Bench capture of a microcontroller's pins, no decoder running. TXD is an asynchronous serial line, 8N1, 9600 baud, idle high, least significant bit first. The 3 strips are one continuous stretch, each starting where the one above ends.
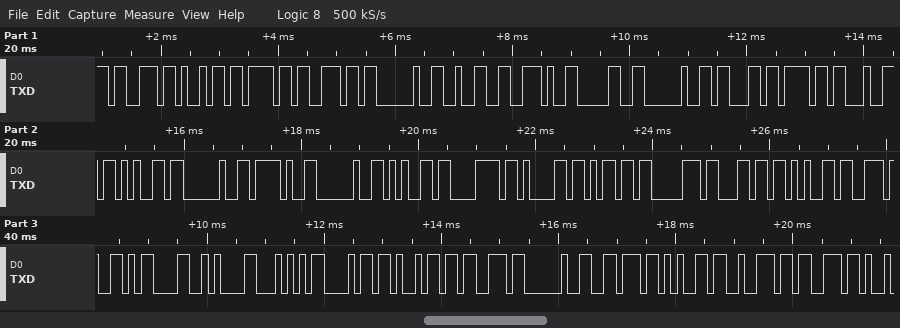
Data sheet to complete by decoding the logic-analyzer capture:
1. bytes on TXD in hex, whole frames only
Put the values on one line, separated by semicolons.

0x73 0x69 0x6F 0x6E 0x20 0x32 0x2E 0x30 0x20 0x63 0x6F 0x64 0x65 0x20 0x2F 0x20 0x65 0x78 0x61 0x6D 0x70 0x6C 0x65 0x2E 0x0D 0x0A 0x54 0x68 0x69 0x73 0x20 0x76 0x65 0x72 0x73
